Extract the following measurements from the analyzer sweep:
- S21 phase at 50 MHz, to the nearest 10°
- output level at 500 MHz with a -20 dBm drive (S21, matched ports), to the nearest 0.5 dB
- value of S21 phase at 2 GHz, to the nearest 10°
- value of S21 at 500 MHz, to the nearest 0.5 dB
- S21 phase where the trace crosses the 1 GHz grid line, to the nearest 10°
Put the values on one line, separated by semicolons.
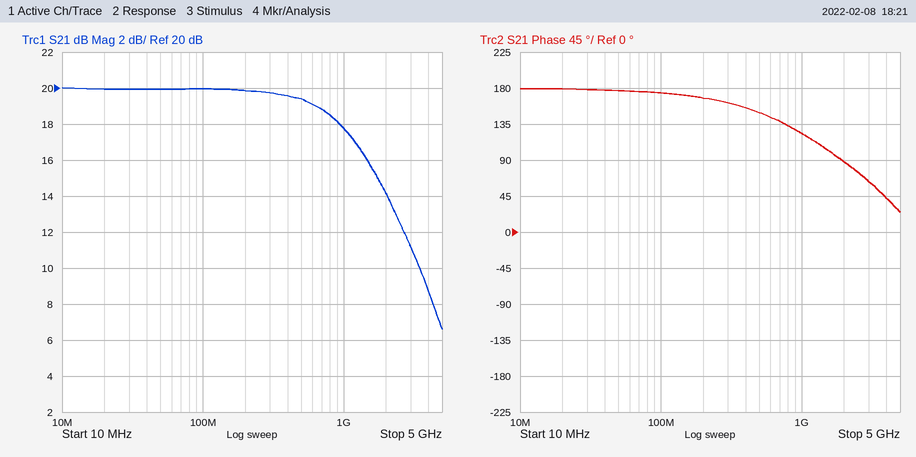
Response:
180°; -0.5 dBm; 90°; 19.5 dB; 120°
